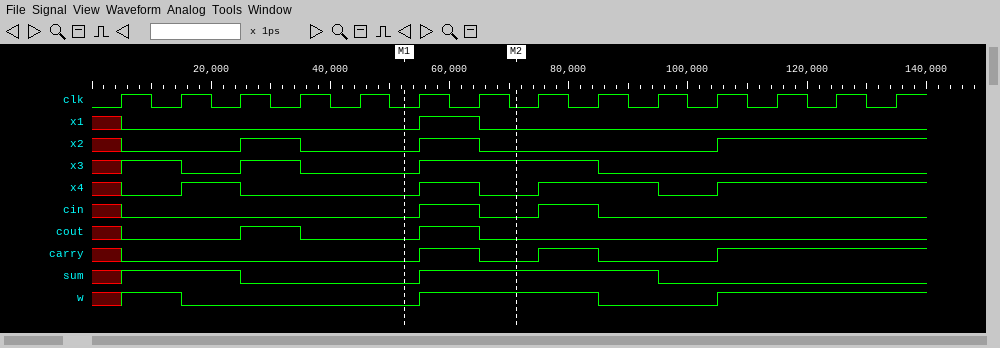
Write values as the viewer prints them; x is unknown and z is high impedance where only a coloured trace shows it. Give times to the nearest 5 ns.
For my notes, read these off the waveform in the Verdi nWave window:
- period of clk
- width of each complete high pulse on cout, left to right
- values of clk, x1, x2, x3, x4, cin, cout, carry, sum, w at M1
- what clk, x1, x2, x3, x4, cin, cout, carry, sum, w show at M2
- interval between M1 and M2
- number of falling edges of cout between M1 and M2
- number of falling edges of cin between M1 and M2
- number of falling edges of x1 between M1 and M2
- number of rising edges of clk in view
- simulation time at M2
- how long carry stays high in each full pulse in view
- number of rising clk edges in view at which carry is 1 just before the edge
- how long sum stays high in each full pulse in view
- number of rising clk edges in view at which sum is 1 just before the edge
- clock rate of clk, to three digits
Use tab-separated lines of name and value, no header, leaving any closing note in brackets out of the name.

period of clk	10 ns
width of each complete high pulse on cout, left to right	10 ns, 10 ns
values of clk, x1, x2, x3, x4, cin, cout, carry, sum, w at M1	clk=0, x1=0, x2=0, x3=0, x4=0, cin=0, cout=0, carry=0, sum=0, w=0
what clk, x1, x2, x3, x4, cin, cout, carry, sum, w show at M2	clk=0, x1=0, x2=0, x3=1, x4=0, cin=0, cout=0, carry=0, sum=1, w=1
interval between M1 and M2	20 ns
number of falling edges of cout between M1 and M2	1
number of falling edges of cin between M1 and M2	1
number of falling edges of x1 between M1 and M2	1
number of rising edges of clk in view	14
simulation time at M2	70 ns
how long carry stays high in each full pulse in view	10 ns, 10 ns
number of rising clk edges in view at which carry is 1 just before the edge	5
how long sum stays high in each full pulse in view	40 ns
number of rising clk edges in view at which sum is 1 just before the edge	6
clock rate of clk, to three digits	100 MHz
